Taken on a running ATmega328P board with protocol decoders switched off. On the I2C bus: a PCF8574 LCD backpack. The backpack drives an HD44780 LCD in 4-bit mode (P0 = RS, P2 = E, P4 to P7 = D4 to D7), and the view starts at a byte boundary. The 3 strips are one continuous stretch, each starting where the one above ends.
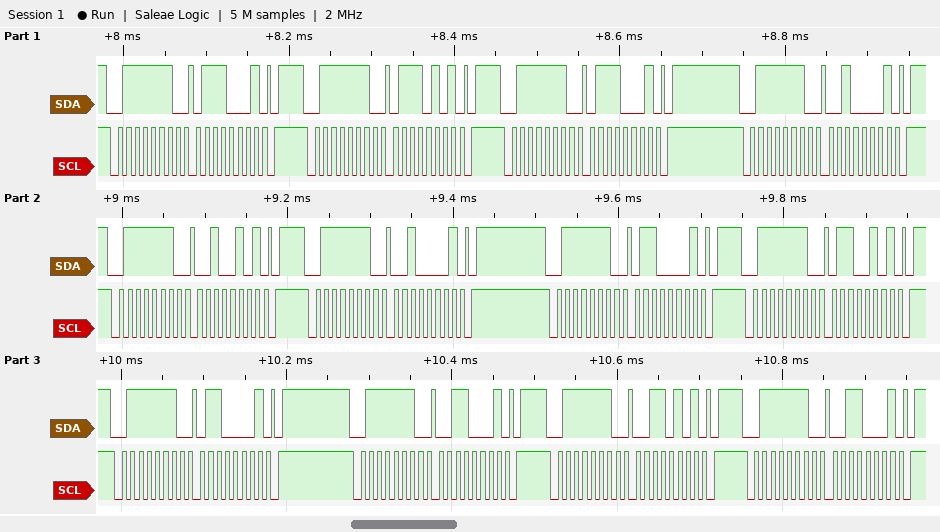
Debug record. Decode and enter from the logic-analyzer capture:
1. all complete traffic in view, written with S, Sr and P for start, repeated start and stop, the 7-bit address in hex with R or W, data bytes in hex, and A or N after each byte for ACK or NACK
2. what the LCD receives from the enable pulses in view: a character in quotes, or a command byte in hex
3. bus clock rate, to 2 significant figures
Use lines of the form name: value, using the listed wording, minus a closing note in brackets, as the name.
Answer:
all complete traffic in view, written with S, Sr and P for start, repeated start and stop, the 7-bit address in hex with R or W, data bytes in hex, and A or N after each byte for ACK or NACK: S 3FW A 71 A P S 3FW A 75 A P S 3FW A 71 A P S 3FW A 21 A P S 3FW A 25 A P S 3FW A 21 A P S 3FW A 61 A P S 3FW A 65 A P S 3FW A 61 A P S 3FW A 31 A P S 3FW A 35 A P S 3FW A 31 A P
what the LCD receives from the enable pulses in view: a character in quotes, or a command byte in hex: 'r' 'c'
bus clock rate, to 2 significant figures: 100 kHz
